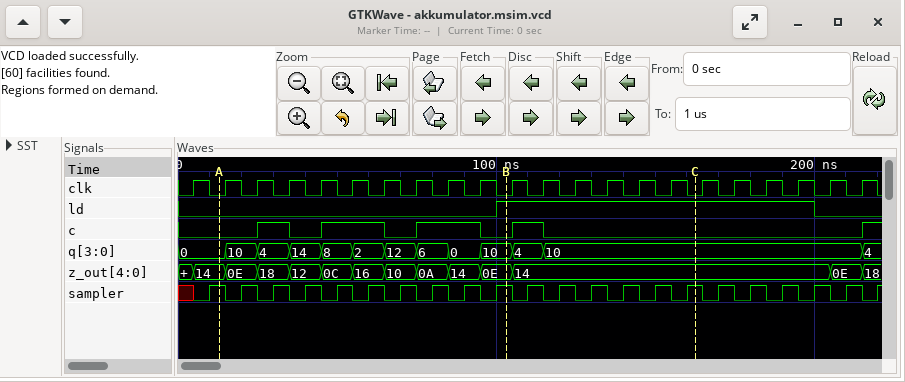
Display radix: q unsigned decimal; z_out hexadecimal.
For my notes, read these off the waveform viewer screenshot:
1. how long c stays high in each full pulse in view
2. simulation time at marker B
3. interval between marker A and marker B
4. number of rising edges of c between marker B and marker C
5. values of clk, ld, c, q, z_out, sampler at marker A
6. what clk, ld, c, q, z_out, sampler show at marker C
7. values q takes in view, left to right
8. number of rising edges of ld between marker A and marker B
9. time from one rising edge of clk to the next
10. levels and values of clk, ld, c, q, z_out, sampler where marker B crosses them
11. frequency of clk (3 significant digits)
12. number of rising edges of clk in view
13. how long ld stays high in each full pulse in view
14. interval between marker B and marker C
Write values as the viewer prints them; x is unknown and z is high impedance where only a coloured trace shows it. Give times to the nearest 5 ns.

10 ns, 20 ns, 20 ns, 10 ns
105 ns
90 ns
1
clk=0, ld=0, c=0, q=0, z_out=14, sampler=1
clk=0, ld=1, c=0, q=10, z_out=14, sampler=1
0, 10, 4, 14, 8, 2, 12, 6, 0, 10, 4, 10, 4
1
10 ns
clk=0, ld=1, c=0, q=10, z_out=0E, sampler=1
100 MHz
22
100 ns
60 ns
